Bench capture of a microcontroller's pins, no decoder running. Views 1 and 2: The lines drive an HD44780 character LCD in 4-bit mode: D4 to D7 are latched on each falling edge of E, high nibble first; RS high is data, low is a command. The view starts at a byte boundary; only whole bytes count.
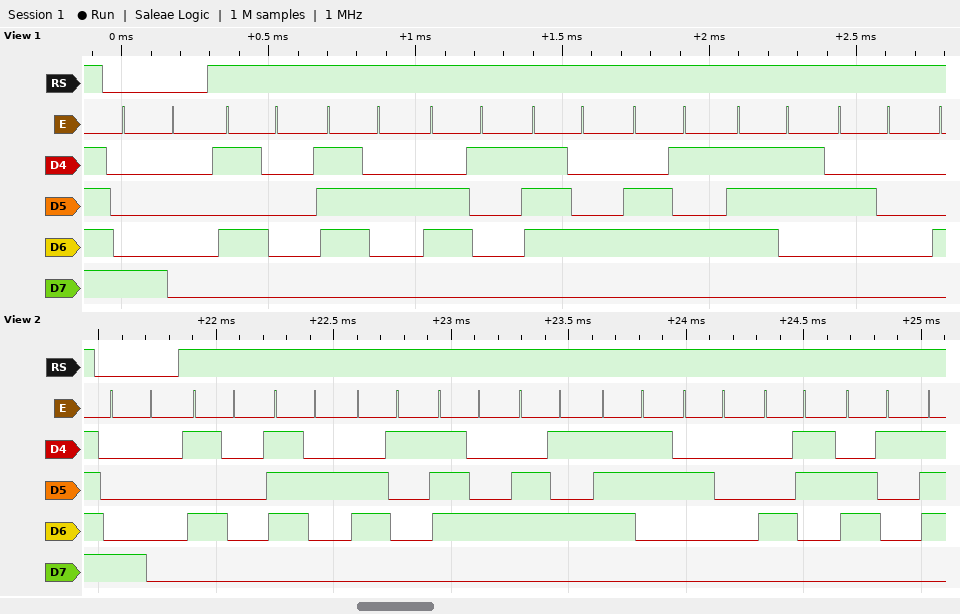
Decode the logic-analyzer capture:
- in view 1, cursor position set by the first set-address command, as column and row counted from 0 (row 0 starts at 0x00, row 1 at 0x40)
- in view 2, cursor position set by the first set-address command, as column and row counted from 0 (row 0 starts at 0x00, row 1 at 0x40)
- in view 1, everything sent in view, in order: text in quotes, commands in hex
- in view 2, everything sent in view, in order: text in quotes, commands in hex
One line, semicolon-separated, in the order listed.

column 0, row 0; column 0, row 0; 0x80 "Prates "; 0x80 "Prates Ca"
